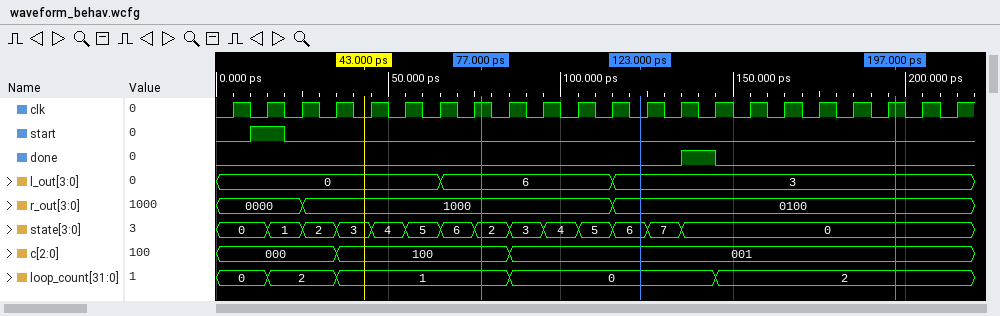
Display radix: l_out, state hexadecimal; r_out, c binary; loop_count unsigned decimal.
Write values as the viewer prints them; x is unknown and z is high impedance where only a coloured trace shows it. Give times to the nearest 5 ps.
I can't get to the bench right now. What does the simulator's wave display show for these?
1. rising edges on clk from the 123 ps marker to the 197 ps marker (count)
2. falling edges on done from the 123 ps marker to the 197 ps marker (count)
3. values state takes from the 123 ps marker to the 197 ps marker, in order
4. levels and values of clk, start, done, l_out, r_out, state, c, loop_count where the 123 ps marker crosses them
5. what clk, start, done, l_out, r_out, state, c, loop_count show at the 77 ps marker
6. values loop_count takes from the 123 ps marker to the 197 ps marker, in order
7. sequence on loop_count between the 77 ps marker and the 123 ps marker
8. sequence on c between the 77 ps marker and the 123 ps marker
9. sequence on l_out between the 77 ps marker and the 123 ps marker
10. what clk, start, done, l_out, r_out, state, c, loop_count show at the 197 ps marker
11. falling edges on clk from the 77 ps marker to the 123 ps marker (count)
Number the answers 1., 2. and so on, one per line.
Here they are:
1. 8
2. 1
3. 6, 7, 0
4. clk=0, start=0, done=0, l_out=3, r_out=0100, state=6, c=001, loop_count=0
5. clk=1, start=0, done=0, l_out=6, r_out=1000, state=2, c=100, loop_count=1
6. 0, 2
7. 1, 0
8. 100, 001
9. 6, 3
10. clk=1, start=0, done=0, l_out=3, r_out=0100, state=0, c=001, loop_count=2
11. 5
